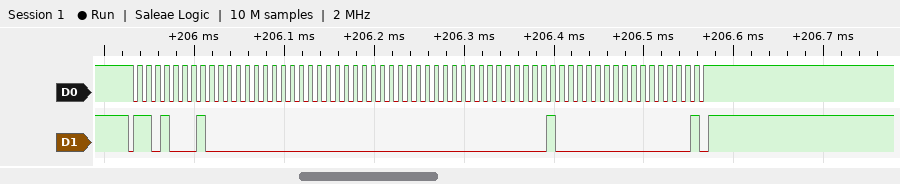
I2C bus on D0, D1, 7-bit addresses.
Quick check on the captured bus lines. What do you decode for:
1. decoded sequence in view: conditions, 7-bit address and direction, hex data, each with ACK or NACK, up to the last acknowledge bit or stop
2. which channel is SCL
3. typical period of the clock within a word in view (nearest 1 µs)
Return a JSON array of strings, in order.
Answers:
["start, address 68 read ACK, 00 ACK, 00 ACK, 00 ACK, 00 ACK, 40 ACK, 00 NACK, stop", "D0", "10 µs"]
